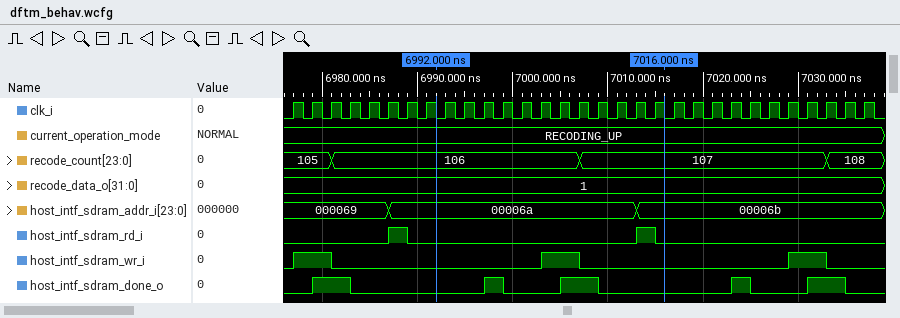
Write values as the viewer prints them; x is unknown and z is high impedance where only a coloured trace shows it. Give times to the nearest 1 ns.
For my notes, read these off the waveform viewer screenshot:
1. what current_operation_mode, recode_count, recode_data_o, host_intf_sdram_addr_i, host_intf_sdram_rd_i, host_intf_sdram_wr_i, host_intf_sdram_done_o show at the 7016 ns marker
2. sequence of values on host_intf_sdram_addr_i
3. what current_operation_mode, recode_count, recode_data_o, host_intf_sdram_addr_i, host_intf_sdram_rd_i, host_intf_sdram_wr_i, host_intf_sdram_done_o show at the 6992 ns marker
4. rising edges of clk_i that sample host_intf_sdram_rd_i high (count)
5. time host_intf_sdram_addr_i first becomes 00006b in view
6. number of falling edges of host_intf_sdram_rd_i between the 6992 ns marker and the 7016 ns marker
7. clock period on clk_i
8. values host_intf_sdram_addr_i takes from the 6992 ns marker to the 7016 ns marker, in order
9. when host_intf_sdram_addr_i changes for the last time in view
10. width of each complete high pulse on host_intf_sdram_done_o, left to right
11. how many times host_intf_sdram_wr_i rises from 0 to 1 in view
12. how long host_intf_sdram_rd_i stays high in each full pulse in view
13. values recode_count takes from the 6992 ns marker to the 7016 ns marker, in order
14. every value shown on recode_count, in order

current_operation_mode=RECODING_UP, recode_count=107, recode_data_o=1, host_intf_sdram_addr_i=00006b, host_intf_sdram_rd_i=0, host_intf_sdram_wr_i=0, host_intf_sdram_done_o=0
000069, 00006a, 00006b
current_operation_mode=RECODING_UP, recode_count=106, recode_data_o=1, host_intf_sdram_addr_i=00006a, host_intf_sdram_rd_i=0, host_intf_sdram_wr_i=0, host_intf_sdram_done_o=0
2
7013 ns
1
2 ns
00006a, 00006b
7013 ns
4 ns, 2 ns, 4 ns, 2 ns, 4 ns
3
2 ns, 2 ns
106, 107
105, 106, 107, 108
